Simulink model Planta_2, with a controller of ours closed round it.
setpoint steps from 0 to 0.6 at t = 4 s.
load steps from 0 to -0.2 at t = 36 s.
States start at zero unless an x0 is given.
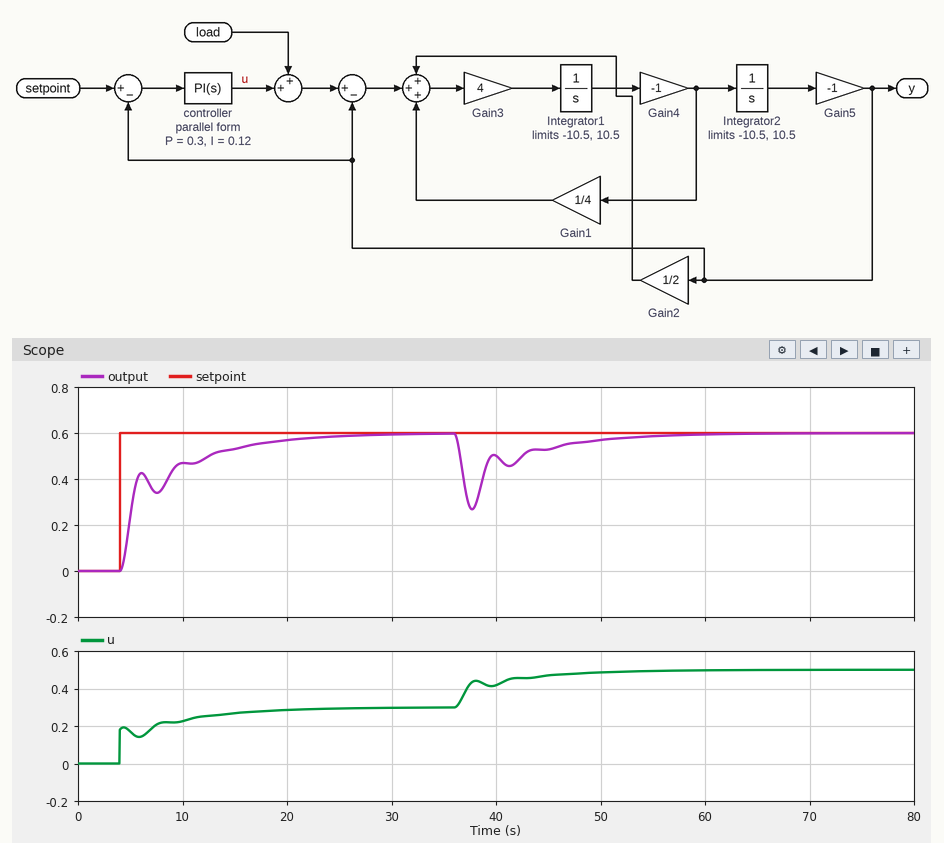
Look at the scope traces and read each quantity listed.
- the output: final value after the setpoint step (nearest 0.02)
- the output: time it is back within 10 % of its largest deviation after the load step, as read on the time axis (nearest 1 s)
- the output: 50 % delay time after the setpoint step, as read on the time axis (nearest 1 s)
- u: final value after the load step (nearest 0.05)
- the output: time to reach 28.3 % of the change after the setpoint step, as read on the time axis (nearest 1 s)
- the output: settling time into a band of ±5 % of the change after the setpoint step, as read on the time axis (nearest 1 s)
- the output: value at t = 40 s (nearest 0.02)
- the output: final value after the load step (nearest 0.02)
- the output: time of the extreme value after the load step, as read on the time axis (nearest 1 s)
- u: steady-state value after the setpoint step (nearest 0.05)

0.60
50 s
5 s
0.50
5 s
20 s
0.50
0.60
38 s
0.30
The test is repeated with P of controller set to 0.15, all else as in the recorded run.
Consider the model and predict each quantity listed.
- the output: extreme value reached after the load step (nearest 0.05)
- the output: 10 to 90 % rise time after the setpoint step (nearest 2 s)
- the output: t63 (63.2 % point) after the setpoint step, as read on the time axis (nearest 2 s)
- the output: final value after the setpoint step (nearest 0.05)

0.20
10 s
8 s
0.60
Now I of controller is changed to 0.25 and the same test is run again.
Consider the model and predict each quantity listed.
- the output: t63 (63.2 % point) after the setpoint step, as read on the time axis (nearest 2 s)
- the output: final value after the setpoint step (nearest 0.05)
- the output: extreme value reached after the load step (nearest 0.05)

6 s
0.60
0.30
